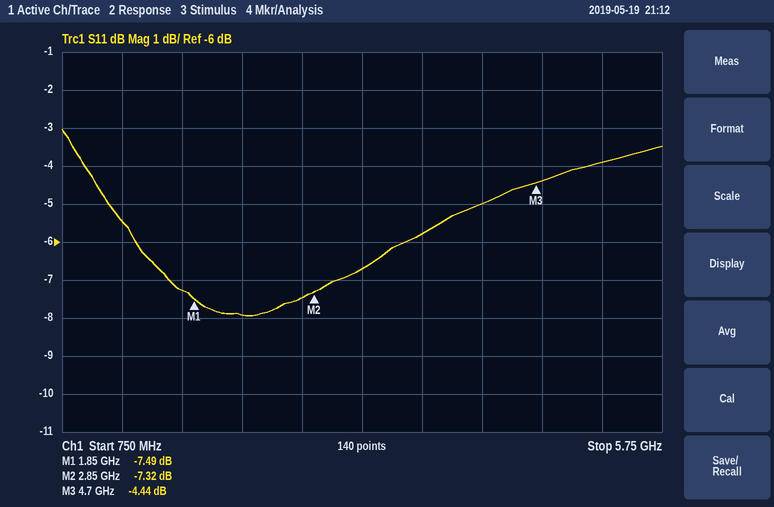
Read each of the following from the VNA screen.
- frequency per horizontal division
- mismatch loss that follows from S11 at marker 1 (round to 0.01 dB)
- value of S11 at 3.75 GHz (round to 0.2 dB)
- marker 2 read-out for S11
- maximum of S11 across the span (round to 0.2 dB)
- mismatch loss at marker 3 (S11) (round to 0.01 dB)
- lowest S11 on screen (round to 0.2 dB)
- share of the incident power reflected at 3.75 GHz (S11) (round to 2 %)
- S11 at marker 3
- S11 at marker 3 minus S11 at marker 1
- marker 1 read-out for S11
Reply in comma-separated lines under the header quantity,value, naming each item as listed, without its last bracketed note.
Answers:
quantity,value
frequency per horizontal division,500 MHz
mismatch loss that follows from S11 at marker 1,0.85 dB
value of S11 at 3.75 GHz,-5.8 dB
marker 2 read-out for S11,-7.32 dB
maximum of S11 across the span,-3.0 dB
mismatch loss at marker 3 (S11),1.94 dB
lowest S11 on screen,-8.0 dB
share of the incident power reflected at 3.75 GHz (S11),26 %
S11 at marker 3,-4.44 dB
S11 at marker 3 minus S11 at marker 1,3.05 dB
marker 1 read-out for S11,-7.49 dB
